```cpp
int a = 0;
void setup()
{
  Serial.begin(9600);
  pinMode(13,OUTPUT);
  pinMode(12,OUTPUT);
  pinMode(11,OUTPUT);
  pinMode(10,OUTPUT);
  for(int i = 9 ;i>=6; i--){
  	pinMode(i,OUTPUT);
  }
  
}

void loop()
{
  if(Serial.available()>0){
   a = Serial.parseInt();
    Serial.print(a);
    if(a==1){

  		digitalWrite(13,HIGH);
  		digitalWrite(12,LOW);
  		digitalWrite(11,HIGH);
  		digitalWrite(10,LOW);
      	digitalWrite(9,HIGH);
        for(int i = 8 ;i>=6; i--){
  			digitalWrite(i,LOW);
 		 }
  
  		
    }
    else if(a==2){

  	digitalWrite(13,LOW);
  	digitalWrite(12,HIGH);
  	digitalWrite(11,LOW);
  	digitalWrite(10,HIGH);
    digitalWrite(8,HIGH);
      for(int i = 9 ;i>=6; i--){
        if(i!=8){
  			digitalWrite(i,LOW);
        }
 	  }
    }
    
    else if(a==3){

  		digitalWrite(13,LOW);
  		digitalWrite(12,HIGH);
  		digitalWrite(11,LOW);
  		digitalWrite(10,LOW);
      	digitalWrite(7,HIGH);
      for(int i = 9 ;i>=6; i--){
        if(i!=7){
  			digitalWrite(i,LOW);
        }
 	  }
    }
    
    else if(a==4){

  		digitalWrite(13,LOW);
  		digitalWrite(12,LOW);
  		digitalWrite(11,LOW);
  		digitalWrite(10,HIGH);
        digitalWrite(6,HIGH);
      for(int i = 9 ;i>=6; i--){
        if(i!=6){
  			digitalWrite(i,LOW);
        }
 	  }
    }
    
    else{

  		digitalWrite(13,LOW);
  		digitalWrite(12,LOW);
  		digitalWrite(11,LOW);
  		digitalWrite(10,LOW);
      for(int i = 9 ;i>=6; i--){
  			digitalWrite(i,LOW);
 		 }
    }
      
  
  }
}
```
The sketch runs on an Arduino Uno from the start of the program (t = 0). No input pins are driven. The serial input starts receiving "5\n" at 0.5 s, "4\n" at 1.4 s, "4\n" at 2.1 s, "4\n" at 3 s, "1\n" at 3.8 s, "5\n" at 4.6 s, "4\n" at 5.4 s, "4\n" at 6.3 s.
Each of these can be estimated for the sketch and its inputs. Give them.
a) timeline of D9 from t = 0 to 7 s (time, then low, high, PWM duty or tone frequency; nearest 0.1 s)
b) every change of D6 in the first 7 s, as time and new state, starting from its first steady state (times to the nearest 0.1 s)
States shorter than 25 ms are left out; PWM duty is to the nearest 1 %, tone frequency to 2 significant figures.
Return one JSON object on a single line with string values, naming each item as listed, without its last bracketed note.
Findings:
{"timeline of D9 from t = 0 to 7 s": "0 s low; 3.8 s high; 4.6 s low", "every change of D6 in the first 7 s, as time and new state, starting from its first steady state": "0 s low; 1.4 s high; 3.8 s low; 5.4 s high"}
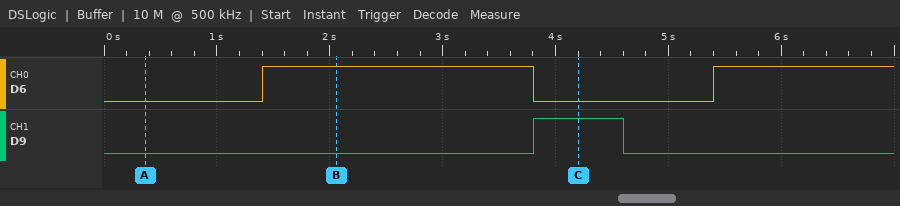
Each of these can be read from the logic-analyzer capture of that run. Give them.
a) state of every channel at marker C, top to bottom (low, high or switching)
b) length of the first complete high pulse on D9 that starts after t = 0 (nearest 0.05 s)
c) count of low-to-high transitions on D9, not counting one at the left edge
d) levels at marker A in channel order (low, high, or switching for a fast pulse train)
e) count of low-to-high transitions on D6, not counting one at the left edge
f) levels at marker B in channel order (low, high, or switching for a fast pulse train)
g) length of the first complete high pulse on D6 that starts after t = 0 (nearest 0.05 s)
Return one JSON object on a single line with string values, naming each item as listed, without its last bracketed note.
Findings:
{"state of every channel at marker C, top to bottom": "D6 low, D9 high", "length of the first complete high pulse on D9 that starts after t = 0": "0.80 s", "count of low-to-high transitions on D9, not counting one at the left edge": "1", "levels at marker A in channel order": "D6 low, D9 low", "count of low-to-high transitions on D6, not counting one at the left edge": "2", "levels at marker B in channel order": "D6 high, D9 low", "length of the first complete high pulse on D6 that starts after t = 0": "2.40 s"}
